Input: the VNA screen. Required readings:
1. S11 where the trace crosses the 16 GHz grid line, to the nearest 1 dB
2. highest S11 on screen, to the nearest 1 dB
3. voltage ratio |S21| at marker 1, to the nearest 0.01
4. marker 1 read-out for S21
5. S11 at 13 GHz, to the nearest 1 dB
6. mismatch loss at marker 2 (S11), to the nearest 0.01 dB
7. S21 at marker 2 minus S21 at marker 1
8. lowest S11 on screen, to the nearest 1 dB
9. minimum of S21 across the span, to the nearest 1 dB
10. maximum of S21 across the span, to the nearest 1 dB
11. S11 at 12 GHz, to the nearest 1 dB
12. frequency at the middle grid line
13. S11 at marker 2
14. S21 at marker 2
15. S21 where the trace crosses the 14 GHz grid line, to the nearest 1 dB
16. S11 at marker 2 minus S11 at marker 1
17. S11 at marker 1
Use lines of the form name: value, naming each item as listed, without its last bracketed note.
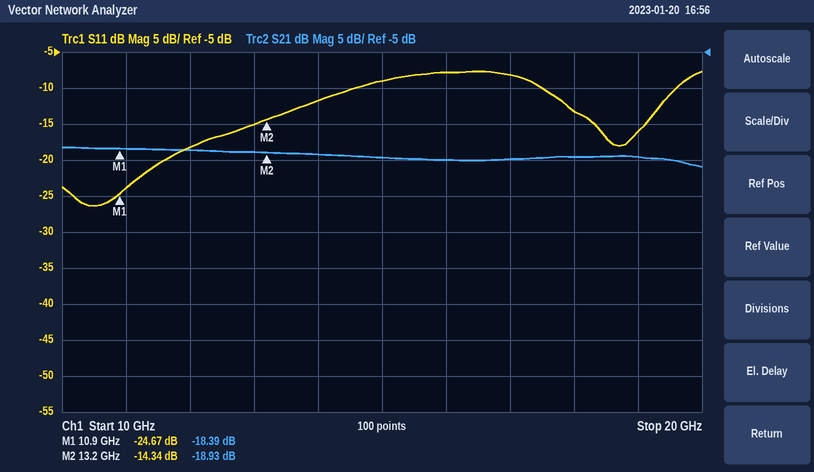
S11 where the trace crosses the 16 GHz grid line, to the nearest 1 dB: -8 dB
highest S11 on screen, to the nearest 1 dB: -8 dB
voltage ratio |S21| at marker 1, to the nearest 0.01: 0.12
marker 1 read-out for S21: -18.39 dB
S11 at 13 GHz, to the nearest 1 dB: -15 dB
mismatch loss at marker 2 (S11), to the nearest 0.01 dB: 0.16 dB
S21 at marker 2 minus S21 at marker 1: -0.54 dB
lowest S11 on screen, to the nearest 1 dB: -26 dB
minimum of S21 across the span, to the nearest 1 dB: -21 dB
maximum of S21 across the span, to the nearest 1 dB: -18 dB
S11 at 12 GHz, to the nearest 1 dB: -18 dB
frequency at the middle grid line: 15 GHz
S11 at marker 2: -14.34 dB
S21 at marker 2: -18.93 dB
S21 where the trace crosses the 14 GHz grid line, to the nearest 1 dB: -19 dB
S11 at marker 2 minus S11 at marker 1: 10.33 dB
S11 at marker 1: -24.67 dB
